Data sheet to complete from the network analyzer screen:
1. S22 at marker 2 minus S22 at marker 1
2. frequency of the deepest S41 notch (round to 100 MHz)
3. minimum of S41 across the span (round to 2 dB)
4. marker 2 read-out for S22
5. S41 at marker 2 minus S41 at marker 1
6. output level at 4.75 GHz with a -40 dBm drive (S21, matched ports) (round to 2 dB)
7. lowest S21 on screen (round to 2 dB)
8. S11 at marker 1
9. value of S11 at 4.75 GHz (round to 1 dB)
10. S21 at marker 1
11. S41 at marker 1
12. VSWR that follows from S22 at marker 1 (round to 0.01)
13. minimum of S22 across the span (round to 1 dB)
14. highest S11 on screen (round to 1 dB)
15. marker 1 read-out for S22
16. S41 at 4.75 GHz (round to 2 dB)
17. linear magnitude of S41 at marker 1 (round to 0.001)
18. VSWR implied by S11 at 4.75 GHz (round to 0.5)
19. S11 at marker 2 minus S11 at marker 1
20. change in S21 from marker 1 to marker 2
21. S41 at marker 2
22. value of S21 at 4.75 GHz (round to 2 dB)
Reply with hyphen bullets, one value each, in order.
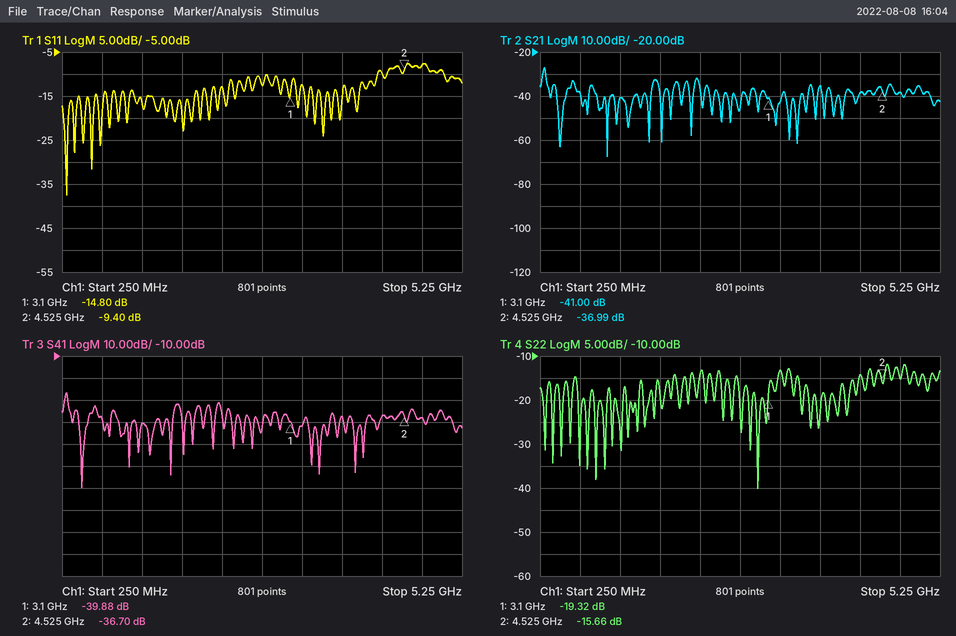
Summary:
- 3.66 dB
- 500 MHz
- -70 dB
- -15.66 dB
- 3.18 dB
- -78 dBm
- -68 dB
- -14.80 dB
- -8 dB
- -41.00 dB
- -39.88 dB
- 1.24
- -40 dB
- -8 dB
- -19.32 dB
- -38 dB
- 0.010
- 2.5
- 5.40 dB
- 4.01 dB
- -36.70 dB
- -38 dB
